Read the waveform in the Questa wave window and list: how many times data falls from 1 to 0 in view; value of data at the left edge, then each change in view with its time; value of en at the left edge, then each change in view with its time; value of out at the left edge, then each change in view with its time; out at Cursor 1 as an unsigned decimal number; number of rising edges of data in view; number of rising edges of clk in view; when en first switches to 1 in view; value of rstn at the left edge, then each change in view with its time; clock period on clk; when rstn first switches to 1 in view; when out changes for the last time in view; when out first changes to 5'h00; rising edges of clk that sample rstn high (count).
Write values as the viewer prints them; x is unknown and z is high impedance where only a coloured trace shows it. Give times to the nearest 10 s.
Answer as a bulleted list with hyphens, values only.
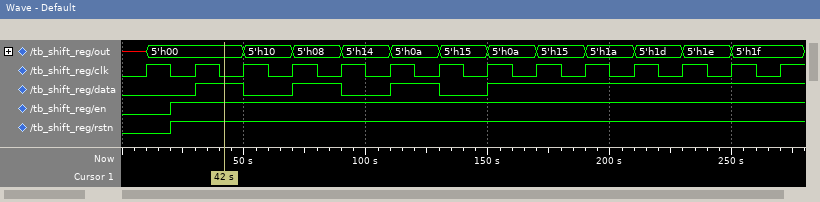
- 3
- 0, 1 at 30 s, 0 at 50 s, 1 at 70 s, 0 at 90 s, 1 at 110 s, 0 at 130 s, 1 at 150 s
- 0, 1 at 20 s
- x, 5'h00 at 10 s, 5'h10 at 50 s, 5'h08 at 70 s, 5'h14 at 90 s, 5'h0a at 110 s, 5'h15 at 130 s, 5'h0a at 150 s, 5'h15 at 170 s, 5'h1a at 190 s, 5'h1d at 210 s, 5'h1e at 230 s, 5'h1f at 250 s
- 0
- 4
- 14
- 20 s
- 0, 1 at 20 s
- 20 s
- 20 s
- 250 s
- 10 s
- 13
